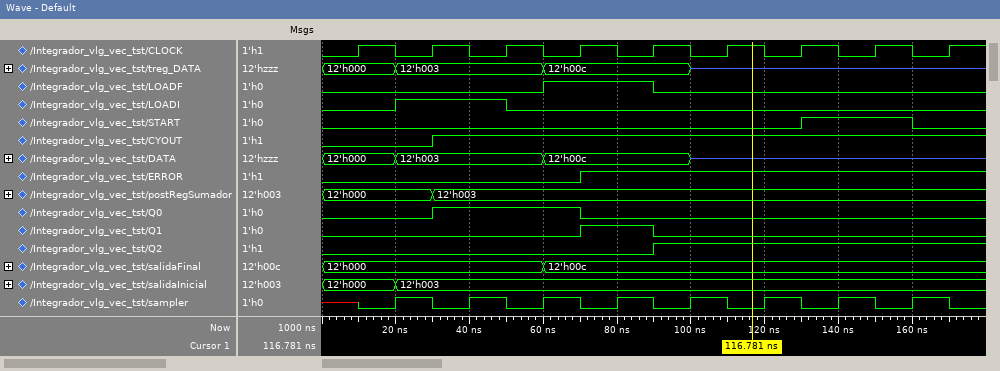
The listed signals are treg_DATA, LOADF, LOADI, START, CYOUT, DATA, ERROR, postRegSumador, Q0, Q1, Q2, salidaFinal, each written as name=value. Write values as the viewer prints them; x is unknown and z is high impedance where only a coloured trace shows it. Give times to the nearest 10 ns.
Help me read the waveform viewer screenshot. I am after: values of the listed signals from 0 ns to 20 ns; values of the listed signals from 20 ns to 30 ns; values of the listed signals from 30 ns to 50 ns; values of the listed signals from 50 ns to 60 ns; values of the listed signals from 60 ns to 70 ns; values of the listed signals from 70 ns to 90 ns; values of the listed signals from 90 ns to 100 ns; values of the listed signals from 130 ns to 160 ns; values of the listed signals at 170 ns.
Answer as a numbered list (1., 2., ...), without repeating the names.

1. treg_DATA=12'h000, LOADF=0, LOADI=0, START=0, CYOUT=0, DATA=12'h000, ERROR=0, postRegSumador=12'h000, Q0=0, Q1=0, Q2=0, salidaFinal=12'h000
2. treg_DATA=12'h003, LOADF=0, LOADI=1, START=0, CYOUT=0, DATA=12'h003, ERROR=0, postRegSumador=12'h000, Q0=0, Q1=0, Q2=0, salidaFinal=12'h000
3. treg_DATA=12'h003, LOADF=0, LOADI=1, START=0, CYOUT=1, DATA=12'h003, ERROR=0, postRegSumador=12'h003, Q0=1, Q1=0, Q2=0, salidaFinal=12'h000
4. treg_DATA=12'h003, LOADF=0, LOADI=0, START=0, CYOUT=1, DATA=12'h003, ERROR=0, postRegSumador=12'h003, Q0=1, Q1=0, Q2=0, salidaFinal=12'h000
5. treg_DATA=12'h00c, LOADF=1, LOADI=0, START=0, CYOUT=1, DATA=12'h00c, ERROR=0, postRegSumador=12'h003, Q0=1, Q1=0, Q2=0, salidaFinal=12'h00c
6. treg_DATA=12'h00c, LOADF=1, LOADI=0, START=0, CYOUT=1, DATA=12'h00c, ERROR=1, postRegSumador=12'h003, Q0=0, Q1=1, Q2=0, salidaFinal=12'h00c
7. treg_DATA=12'h00c, LOADF=0, LOADI=0, START=0, CYOUT=1, DATA=12'h00c, ERROR=1, postRegSumador=12'h003, Q0=0, Q1=0, Q2=1, salidaFinal=12'h00c
8. treg_DATA=z, LOADF=0, LOADI=0, START=1, CYOUT=1, DATA=z, ERROR=1, postRegSumador=12'h003, Q0=0, Q1=0, Q2=1, salidaFinal=12'h00c
9. treg_DATA=z, LOADF=0, LOADI=0, START=0, CYOUT=1, DATA=z, ERROR=1, postRegSumador=12'h003, Q0=0, Q1=0, Q2=1, salidaFinal=12'h00c
